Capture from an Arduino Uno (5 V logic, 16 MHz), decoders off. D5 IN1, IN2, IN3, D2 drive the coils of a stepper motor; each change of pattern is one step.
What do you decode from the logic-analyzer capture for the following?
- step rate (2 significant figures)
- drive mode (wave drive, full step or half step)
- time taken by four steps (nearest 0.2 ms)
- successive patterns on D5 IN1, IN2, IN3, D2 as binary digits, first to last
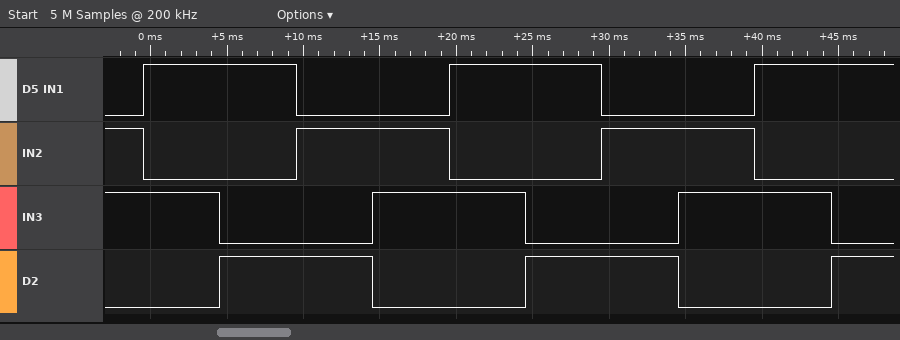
200 steps/s
full step
20.0 ms
0110 1010 1001 0101 0110 1010 1001 0101 0110 1010 1001
